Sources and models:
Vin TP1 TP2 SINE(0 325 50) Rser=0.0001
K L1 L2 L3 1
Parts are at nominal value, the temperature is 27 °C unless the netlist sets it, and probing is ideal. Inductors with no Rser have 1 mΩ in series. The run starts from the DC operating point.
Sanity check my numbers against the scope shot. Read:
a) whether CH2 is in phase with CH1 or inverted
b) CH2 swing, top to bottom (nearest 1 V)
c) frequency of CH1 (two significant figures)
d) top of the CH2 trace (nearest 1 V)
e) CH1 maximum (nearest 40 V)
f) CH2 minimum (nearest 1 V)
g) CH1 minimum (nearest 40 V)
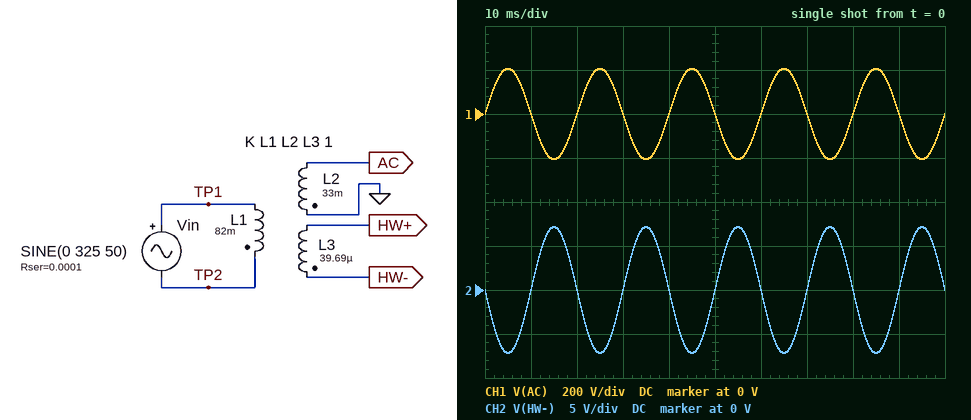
inverted
14 V
50 Hz
7 V
200 V
-7 V
-200 V
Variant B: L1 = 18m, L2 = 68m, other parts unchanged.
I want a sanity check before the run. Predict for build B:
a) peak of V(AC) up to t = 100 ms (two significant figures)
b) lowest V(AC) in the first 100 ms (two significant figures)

630 V
-630 V
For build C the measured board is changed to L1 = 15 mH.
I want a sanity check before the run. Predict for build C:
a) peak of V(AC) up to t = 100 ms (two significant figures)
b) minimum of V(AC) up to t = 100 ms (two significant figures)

480 V
-480 V
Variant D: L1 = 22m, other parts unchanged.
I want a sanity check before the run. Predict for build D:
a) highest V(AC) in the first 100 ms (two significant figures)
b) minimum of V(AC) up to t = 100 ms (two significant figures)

400 V
-400 V
